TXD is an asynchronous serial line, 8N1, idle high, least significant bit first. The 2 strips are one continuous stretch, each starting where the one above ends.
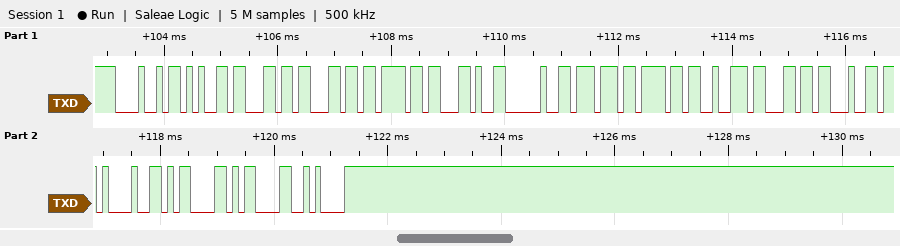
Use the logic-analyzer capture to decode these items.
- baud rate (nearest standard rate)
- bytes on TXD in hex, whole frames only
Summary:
9600 baud
48 65 6C 6C 6F 2C 20 77 6F 72 6C 64 21 0D 0D 0A
